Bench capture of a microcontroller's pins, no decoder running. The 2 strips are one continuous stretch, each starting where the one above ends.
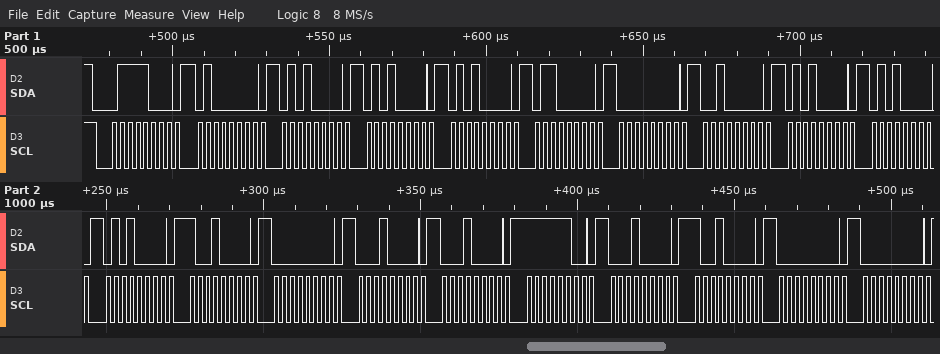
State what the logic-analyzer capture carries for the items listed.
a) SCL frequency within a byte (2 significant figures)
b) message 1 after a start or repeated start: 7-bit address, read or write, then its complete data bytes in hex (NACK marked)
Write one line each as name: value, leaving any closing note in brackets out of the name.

SCL frequency within a byte: 400 kHz
message 1 after a start or repeated start: 7-bit address, read or write, then its complete data bytes in hex: 0x3C write: 40 50 50 50 60 00 20 50 50 50 90 00 10 10 FC 10 90 00 00
